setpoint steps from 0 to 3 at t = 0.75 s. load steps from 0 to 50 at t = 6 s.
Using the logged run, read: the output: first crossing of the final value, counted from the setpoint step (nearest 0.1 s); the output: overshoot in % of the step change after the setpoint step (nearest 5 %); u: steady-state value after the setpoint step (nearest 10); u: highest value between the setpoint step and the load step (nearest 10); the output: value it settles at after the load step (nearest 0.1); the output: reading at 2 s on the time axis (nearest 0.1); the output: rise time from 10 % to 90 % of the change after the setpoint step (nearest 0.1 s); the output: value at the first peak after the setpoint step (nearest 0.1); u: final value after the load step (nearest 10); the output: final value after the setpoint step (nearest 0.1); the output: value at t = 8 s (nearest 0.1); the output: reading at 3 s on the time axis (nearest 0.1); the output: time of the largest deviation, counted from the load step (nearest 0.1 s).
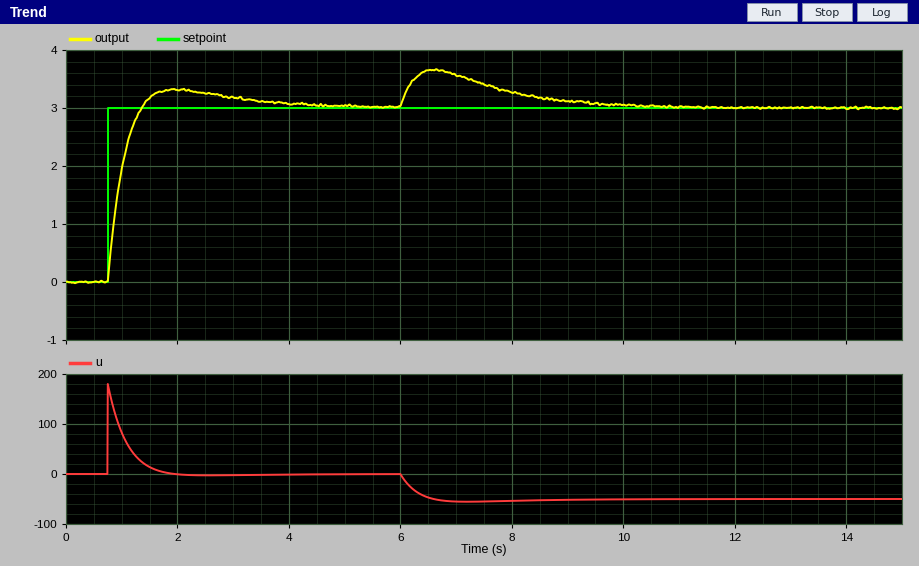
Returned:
0.6 s
10 %
0
180
3.0
3.3
0.4 s
3.3
-50
3.0
3.3
3.2
0.6 s
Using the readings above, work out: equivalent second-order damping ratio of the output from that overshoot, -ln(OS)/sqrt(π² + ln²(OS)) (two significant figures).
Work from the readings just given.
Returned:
0.59
